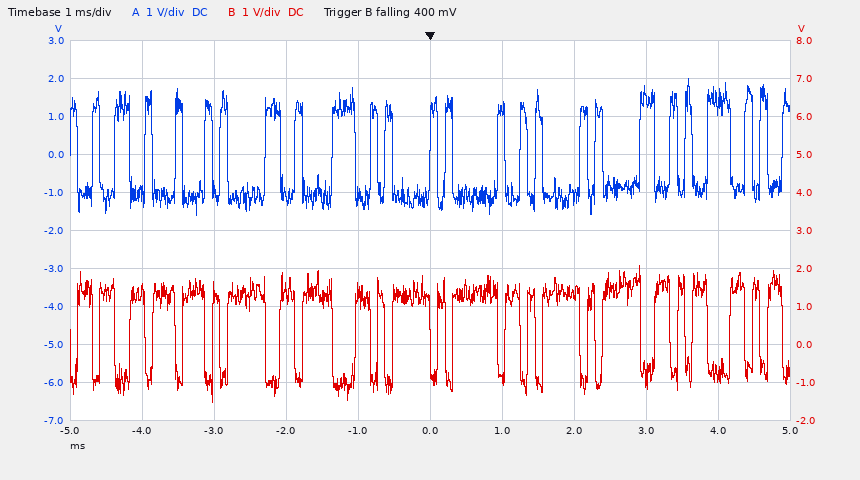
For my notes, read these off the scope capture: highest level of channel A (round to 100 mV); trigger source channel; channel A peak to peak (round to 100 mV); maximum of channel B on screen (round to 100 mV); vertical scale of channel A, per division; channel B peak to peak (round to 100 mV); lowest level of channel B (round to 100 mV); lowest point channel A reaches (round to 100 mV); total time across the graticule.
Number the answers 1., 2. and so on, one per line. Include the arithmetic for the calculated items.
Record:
1. 2.0 V
2. channel B
3. 2.0 V − (-1.6 V) = 3.6 V
4. 2.1 V
5. 1 V
6. 2.1 V − (-1.5 V) = 3.6 V
7. -1.5 V
8. -1.6 V
9. 10 ms
